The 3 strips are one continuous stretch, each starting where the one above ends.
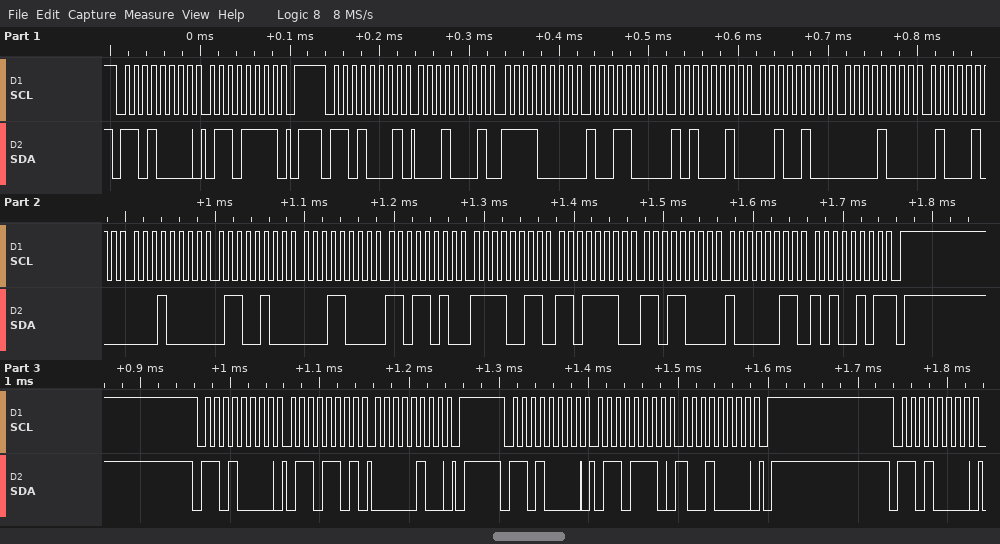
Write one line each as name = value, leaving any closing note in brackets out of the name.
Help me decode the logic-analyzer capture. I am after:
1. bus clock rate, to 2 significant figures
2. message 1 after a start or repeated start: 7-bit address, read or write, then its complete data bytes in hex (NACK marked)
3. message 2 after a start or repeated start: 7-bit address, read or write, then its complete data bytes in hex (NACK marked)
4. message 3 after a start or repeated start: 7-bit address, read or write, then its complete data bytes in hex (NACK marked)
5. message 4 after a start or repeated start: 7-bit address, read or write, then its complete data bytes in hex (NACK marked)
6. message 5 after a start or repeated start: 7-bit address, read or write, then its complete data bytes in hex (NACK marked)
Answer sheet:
bus clock rate, to 2 significant figures = 100 kHz
message 1 after a start or repeated start: 7-bit address, read or write, then its complete data bytes in hex = 0x68 write: 6F
message 2 after a start or repeated start: 7-bit address, read or write, then its complete data bytes in hex = 0x68 read: 11 F0 98 A2 24 08 44 10 64 18 DA F3 DE D8 83 A5 NACK
message 3 after a start or repeated start: 7-bit address, read or write, then its complete data bytes in hex = 0x68 write: 6D 04
message 4 after a start or repeated start: 7-bit address, read or write, then its complete data bytes in hex = 0x68 write: 6E 90
message 5 after a start or repeated start: 7-bit address, read or write, then its complete data bytes in hex = 0x68 write
